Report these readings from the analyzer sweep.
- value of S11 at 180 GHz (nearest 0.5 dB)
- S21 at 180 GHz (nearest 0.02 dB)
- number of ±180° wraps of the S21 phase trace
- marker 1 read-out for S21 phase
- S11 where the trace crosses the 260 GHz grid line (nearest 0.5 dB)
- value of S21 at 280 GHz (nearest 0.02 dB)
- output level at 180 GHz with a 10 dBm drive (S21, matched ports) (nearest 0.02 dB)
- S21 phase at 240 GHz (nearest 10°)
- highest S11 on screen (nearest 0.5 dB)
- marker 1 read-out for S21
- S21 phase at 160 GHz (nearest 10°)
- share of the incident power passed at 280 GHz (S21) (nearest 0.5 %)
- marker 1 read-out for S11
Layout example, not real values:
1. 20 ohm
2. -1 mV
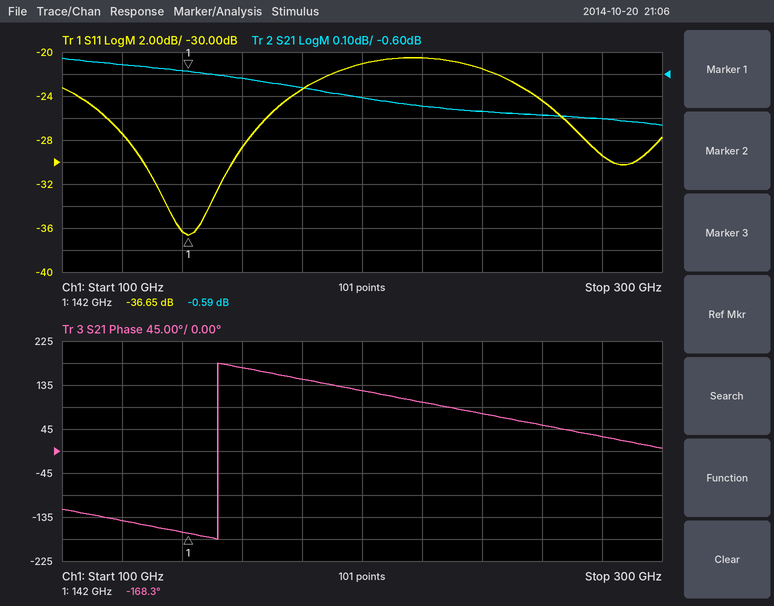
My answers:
1. -23.5 dB
2. -0.66 dB
3. 1
4. -168.3°
5. -24.5 dB
6. -0.80 dB
7. 9.34 dBm
8. 80°
9. -20.5 dB
10. -0.59 dB
11. 170°
12. 83.0 %
13. -36.65 dB
